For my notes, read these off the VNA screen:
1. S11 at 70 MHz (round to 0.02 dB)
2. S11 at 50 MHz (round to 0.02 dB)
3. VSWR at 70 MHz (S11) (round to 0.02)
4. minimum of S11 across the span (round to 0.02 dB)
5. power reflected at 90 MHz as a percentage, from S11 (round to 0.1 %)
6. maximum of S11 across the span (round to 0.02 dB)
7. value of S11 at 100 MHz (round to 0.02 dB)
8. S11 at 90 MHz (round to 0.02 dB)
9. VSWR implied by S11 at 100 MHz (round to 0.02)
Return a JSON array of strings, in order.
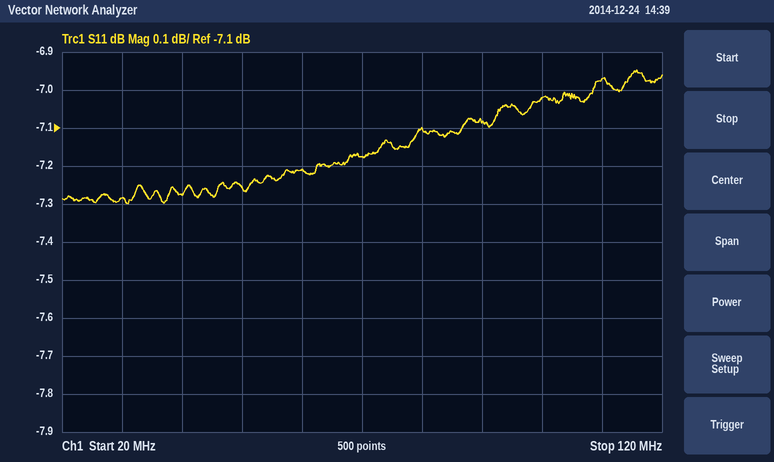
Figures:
["-7.18 dB", "-7.26 dB", "2.56", "-7.30 dB", "19.6 %", "-6.94 dB", "-7.02 dB", "-7.08 dB", "2.60"]
